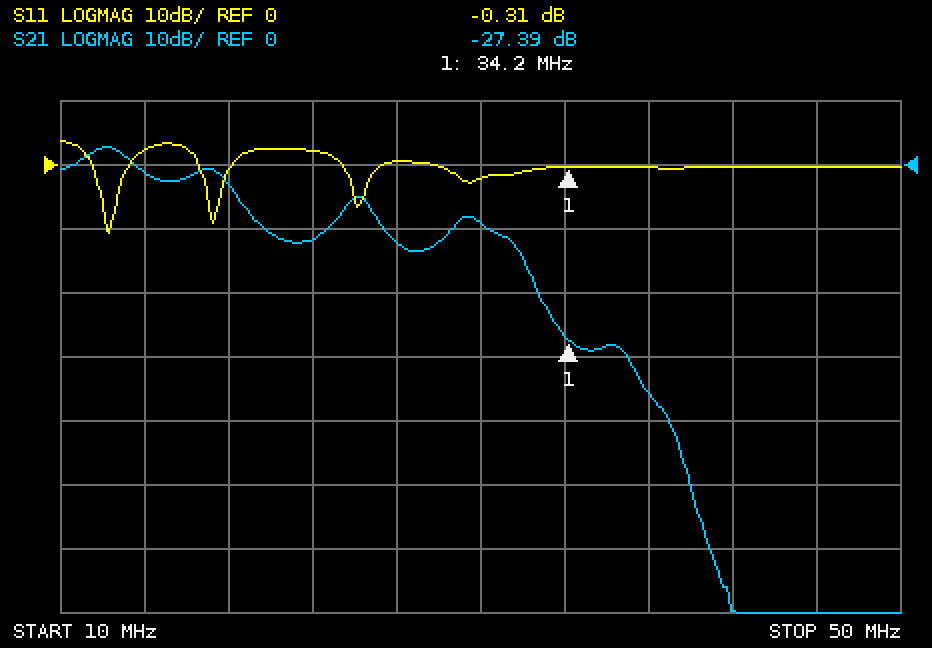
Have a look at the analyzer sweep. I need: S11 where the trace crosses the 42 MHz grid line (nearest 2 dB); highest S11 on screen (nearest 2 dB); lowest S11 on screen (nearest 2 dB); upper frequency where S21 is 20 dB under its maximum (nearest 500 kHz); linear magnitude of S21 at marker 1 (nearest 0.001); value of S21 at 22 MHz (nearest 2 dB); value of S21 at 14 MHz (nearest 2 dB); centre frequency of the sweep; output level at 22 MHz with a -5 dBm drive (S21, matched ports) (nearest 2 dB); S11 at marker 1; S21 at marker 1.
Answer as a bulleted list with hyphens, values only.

- 0 dB
- 4 dB
- -10 dB
- 32.5 MHz
- 0.043
- -12 dB
- -2 dB
- 30 MHz
- -16 dBm
- -0.31 dB
- -27.39 dB
